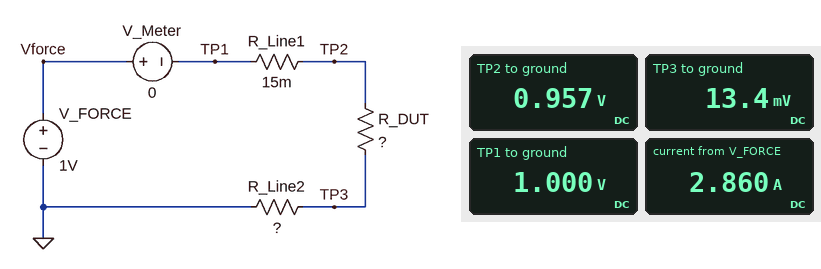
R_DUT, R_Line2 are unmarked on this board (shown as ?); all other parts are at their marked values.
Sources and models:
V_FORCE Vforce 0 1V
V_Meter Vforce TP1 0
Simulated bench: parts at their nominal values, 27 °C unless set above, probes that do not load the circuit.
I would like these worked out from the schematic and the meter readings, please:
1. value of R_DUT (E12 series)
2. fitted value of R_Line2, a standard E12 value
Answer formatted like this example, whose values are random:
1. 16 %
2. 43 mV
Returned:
1. 0.33 Ω
2. 4.7 mΩ
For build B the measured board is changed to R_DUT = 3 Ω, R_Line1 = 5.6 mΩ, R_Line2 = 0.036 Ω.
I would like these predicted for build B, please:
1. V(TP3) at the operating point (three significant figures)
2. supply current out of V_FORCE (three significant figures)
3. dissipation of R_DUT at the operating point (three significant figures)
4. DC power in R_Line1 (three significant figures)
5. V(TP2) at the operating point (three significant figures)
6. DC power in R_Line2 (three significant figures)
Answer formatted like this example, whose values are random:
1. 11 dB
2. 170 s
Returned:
1. 11.8 mV
2. 329 mA
3. 324 mW
4. 605 µW
5. 998 mV
6. 3.89 mW
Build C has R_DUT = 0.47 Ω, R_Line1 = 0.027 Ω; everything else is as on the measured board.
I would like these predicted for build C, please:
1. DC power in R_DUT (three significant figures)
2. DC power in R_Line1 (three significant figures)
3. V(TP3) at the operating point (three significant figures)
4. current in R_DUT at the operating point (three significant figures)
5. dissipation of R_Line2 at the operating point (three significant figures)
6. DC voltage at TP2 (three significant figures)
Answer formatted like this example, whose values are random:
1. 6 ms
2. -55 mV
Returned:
1. 1.87 W
2. 107 mW
3. 9.37 mV
4. 1.99 A
5. 18.7 mW
6. 946 mV
